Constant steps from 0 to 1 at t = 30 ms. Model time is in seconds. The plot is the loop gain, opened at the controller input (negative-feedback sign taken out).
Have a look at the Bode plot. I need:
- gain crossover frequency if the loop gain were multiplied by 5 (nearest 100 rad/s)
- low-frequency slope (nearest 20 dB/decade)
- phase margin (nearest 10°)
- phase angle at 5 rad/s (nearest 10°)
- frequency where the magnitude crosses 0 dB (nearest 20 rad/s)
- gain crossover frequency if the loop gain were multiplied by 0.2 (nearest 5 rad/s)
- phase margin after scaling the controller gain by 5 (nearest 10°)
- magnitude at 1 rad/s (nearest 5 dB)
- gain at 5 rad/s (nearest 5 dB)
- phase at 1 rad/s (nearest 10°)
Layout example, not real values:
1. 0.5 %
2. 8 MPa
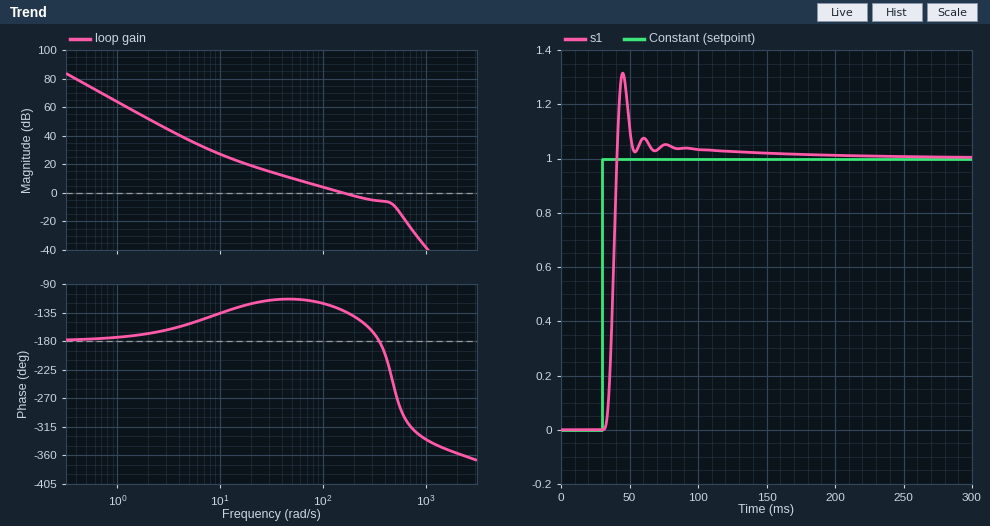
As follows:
1. 600 rad/s
2. -40 dB/decade
3. 50°
4. -150°
5. 160 rad/s
6. 35 rad/s
7. -100°
8. 65 dB
9. 35 dB
10. -170°
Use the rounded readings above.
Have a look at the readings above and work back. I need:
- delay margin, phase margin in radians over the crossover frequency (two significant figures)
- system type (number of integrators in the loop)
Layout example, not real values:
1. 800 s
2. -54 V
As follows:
1. 0.0055 s
2. 2
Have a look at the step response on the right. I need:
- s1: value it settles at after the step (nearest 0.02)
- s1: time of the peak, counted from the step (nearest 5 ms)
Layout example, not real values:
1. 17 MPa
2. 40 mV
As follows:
1. 1.00
2. 15 ms
